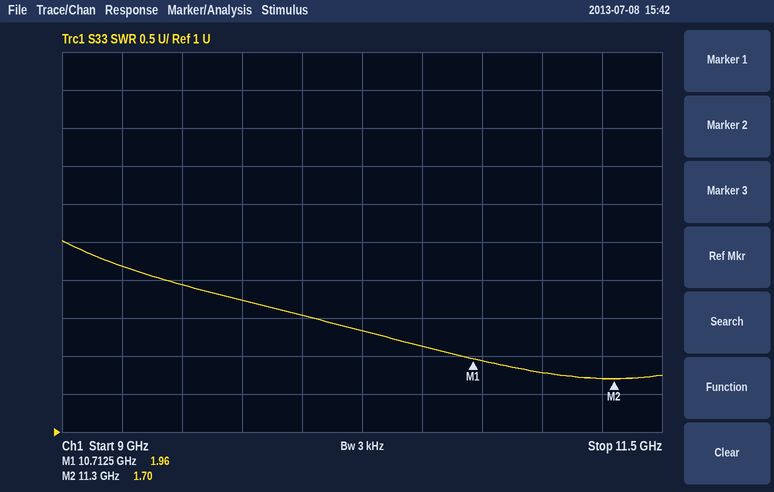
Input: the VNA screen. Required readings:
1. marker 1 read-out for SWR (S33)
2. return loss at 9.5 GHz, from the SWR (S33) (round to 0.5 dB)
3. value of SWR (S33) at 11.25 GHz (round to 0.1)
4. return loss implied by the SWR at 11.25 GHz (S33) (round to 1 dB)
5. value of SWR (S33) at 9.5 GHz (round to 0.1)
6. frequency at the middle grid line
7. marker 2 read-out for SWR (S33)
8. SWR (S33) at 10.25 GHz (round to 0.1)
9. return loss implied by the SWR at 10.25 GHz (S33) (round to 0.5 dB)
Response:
1.96
6.0 dB
1.7
12 dB
2.9
10.25 GHz
1.70
2.3
8.0 dB
